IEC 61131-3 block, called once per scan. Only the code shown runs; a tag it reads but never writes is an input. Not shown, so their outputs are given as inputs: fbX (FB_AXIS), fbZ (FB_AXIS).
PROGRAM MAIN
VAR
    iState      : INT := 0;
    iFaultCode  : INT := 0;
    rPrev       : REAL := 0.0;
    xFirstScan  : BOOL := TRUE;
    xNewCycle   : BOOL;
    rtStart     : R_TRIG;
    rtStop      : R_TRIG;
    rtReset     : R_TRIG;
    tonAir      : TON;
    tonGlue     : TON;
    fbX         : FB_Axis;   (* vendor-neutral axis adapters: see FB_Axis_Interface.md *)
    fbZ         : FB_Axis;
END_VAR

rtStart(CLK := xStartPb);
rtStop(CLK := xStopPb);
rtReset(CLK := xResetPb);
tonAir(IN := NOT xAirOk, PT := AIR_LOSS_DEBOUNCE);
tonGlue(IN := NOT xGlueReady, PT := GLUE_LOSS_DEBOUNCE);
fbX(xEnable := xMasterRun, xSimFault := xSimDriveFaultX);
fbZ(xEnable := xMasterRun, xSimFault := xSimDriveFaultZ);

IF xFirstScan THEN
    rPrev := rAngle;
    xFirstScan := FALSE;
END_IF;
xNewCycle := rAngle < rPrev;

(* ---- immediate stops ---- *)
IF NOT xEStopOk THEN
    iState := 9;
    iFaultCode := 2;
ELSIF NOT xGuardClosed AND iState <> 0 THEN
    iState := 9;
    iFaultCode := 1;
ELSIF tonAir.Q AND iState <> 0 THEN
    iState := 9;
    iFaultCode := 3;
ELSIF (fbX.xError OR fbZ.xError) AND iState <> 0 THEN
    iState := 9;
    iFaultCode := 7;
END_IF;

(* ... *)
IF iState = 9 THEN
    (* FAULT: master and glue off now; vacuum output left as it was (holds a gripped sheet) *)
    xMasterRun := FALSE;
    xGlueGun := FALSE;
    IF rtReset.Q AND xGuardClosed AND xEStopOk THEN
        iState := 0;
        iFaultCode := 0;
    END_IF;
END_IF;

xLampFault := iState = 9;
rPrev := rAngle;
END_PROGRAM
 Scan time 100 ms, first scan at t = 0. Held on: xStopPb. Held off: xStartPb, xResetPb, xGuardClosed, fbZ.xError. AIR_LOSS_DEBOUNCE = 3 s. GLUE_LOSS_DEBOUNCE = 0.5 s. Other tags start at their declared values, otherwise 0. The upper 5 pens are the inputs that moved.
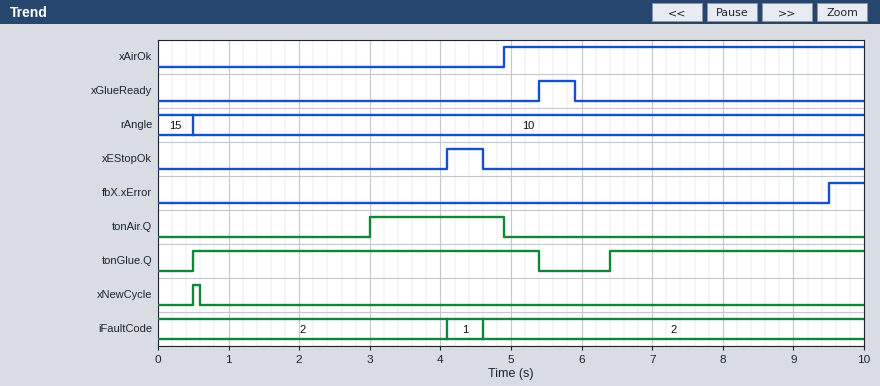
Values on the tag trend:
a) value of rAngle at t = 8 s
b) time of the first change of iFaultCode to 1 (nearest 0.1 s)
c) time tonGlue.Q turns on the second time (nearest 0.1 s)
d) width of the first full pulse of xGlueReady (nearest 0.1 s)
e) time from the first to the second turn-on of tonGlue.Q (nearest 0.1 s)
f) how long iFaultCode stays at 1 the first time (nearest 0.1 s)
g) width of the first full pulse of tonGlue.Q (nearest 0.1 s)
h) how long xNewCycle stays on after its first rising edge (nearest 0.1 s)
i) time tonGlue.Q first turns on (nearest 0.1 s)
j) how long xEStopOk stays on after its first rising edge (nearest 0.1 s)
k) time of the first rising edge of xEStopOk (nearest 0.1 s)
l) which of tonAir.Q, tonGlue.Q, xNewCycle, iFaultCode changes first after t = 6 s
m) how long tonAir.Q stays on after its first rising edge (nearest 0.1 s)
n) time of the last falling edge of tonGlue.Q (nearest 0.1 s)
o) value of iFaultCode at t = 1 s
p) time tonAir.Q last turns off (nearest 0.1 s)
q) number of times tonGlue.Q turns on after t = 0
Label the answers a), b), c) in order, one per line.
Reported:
a) 10
b) 4.1 s
c) 6.4 s
d) 0.5 s
e) 5.9 s
f) 0.5 s
g) 4.9 s
h) 0.1 s
i) 0.5 s
j) 0.5 s
k) 4.1 s
l) tonGlue.Q
m) 1.9 s
n) 5.4 s
o) 2
p) 4.9 s
q) 2
